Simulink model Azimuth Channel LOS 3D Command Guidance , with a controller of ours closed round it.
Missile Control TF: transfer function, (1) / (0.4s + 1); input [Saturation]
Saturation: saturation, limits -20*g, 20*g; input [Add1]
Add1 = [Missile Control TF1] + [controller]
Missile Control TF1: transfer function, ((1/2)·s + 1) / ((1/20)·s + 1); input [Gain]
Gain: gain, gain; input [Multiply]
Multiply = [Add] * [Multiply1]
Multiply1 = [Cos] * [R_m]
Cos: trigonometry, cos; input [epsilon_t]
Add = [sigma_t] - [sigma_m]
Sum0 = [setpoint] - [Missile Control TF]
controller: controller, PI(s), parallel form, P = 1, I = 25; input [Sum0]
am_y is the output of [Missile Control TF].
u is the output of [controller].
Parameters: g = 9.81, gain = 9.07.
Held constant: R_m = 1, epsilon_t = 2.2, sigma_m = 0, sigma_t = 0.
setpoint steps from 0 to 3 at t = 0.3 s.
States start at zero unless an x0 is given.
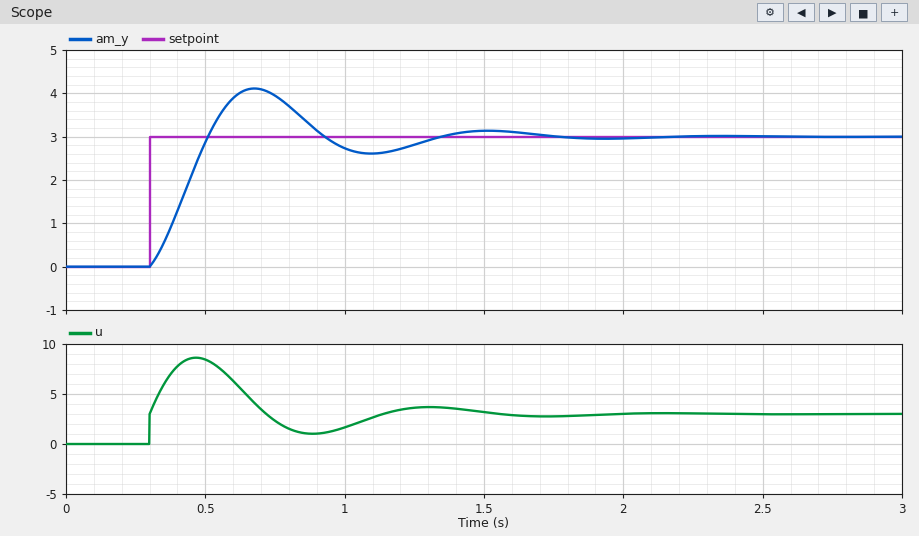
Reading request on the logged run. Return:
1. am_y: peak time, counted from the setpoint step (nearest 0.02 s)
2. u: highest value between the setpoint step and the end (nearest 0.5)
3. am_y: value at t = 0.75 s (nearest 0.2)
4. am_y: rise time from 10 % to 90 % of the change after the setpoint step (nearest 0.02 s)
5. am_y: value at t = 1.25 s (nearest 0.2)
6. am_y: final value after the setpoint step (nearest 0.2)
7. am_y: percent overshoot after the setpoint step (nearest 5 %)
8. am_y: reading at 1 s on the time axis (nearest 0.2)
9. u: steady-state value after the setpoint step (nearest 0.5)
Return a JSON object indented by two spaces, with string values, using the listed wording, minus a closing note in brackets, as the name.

{
  "am_y: peak time, counted from the setpoint step": "0.38 s",
  "u: highest value between the setpoint step and the end": "8.5",
  "am_y: value at t = 0.75 s": "4.0",
  "am_y: rise time from 10 % to 90 % of the change after the setpoint step": "0.16 s",
  "am_y: value at t = 1.25 s": "2.8",
  "am_y: final value after the setpoint step": "3.0",
  "am_y: percent overshoot after the setpoint step": "35 %",
  "am_y: reading at 1 s on the time axis": "2.8",
  "u: steady-state value after the setpoint step": "3.0"
}
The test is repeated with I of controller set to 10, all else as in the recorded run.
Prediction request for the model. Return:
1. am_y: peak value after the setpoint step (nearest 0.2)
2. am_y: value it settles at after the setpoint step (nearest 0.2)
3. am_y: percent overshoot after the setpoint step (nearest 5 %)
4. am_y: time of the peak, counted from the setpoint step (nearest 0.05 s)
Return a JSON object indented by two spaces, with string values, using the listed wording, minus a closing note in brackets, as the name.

{
  "am_y: peak value after the setpoint step": "3.6",
  "am_y: value it settles at after the setpoint step": "3.0",
  "am_y: percent overshoot after the setpoint step": "20 %",
  "am_y: time of the peak, counted from the setpoint step": "0.60 s"
}
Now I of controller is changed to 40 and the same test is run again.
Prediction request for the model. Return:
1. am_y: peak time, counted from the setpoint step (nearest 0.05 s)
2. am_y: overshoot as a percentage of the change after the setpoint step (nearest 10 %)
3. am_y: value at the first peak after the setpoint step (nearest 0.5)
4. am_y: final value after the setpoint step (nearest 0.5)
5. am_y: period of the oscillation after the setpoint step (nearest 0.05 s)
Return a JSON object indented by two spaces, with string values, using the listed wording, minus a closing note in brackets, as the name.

{
  "am_y: peak time, counted from the setpoint step": "0.30 s",
  "am_y: overshoot as a percentage of the change after the setpoint step": "50 %",
  "am_y: value at the first peak after the setpoint step": "4.5",
  "am_y: final value after the setpoint step": "3.0",
  "am_y: period of the oscillation after the setpoint step": "0.65 s"
}
